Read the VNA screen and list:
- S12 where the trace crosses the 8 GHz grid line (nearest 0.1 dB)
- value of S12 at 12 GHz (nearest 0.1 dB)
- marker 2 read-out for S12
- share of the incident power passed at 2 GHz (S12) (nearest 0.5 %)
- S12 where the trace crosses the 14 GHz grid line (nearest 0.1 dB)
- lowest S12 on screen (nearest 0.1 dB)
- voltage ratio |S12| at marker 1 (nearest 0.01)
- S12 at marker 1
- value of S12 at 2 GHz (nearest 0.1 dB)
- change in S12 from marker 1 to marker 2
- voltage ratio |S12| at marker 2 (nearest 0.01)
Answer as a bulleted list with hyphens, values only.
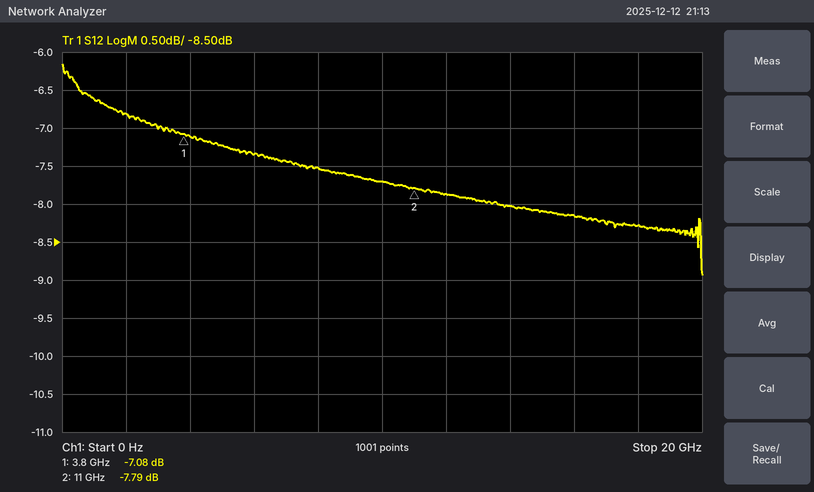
- -7.5 dB
- -7.9 dB
- -7.79 dB
- 21.0 %
- -8.0 dB
- -8.9 dB
- 0.44
- -7.08 dB
- -6.8 dB
- -0.71 dB
- 0.41
